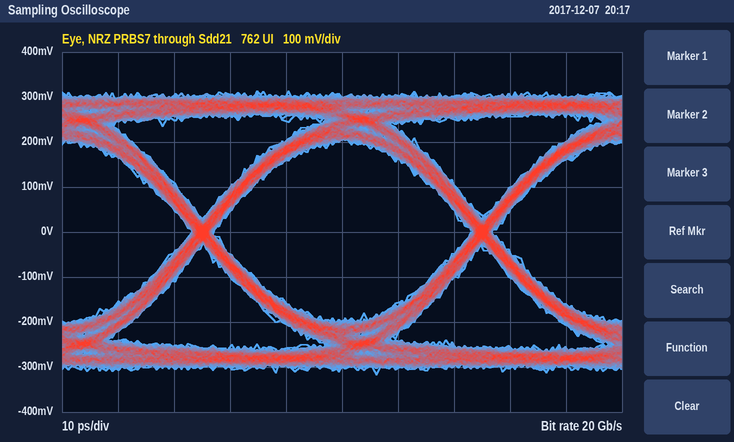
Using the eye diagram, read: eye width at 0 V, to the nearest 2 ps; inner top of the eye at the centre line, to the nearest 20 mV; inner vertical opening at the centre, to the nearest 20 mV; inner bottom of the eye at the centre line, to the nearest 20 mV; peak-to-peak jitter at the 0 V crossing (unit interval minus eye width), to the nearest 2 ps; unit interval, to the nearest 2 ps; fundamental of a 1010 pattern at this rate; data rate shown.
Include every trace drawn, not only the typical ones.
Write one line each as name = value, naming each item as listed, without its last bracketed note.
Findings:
eye width at 0 V, to the nearest 2 ps = 46 ps
inner top of the eye at the centre line, to the nearest 20 mV = 200 mV
inner vertical opening at the centre, to the nearest 20 mV = 400 mV
inner bottom of the eye at the centre line, to the nearest 20 mV = -200 mV
peak-to-peak jitter at the 0 V crossing (unit interval minus eye width), to the nearest 2 ps = 4 ps
unit interval, to the nearest 2 ps = 50 ps
fundamental of a 1010 pattern at this rate = 10 GHz
data rate shown = 20 Gb/s
